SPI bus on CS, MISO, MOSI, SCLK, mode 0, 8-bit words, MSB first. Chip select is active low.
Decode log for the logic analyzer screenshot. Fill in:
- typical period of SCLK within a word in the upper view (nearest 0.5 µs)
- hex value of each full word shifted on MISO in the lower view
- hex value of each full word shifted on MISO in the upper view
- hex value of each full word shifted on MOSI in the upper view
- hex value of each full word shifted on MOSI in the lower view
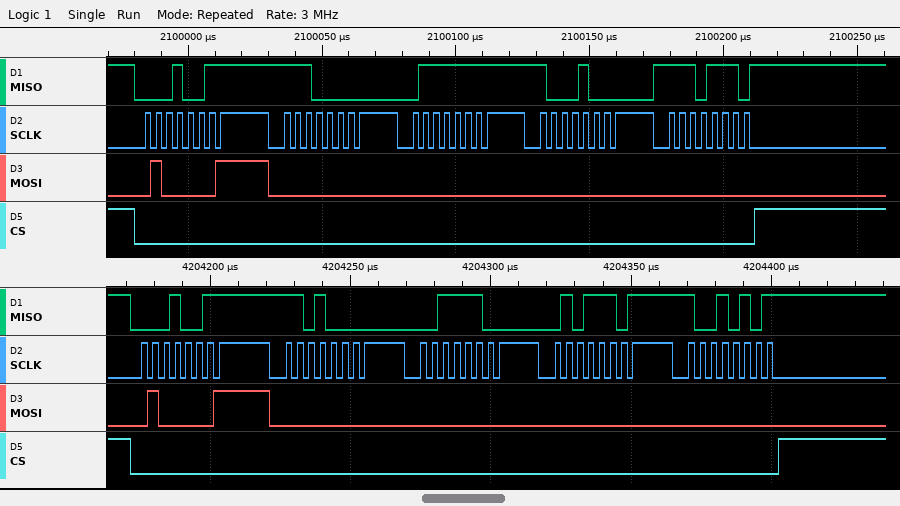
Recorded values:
4 µs
13, D0, 3C, 5D, 95
13, E0, 7F, 88, EE
41, 00, 00, 00, 00
41, 00, 00, 00, 00
